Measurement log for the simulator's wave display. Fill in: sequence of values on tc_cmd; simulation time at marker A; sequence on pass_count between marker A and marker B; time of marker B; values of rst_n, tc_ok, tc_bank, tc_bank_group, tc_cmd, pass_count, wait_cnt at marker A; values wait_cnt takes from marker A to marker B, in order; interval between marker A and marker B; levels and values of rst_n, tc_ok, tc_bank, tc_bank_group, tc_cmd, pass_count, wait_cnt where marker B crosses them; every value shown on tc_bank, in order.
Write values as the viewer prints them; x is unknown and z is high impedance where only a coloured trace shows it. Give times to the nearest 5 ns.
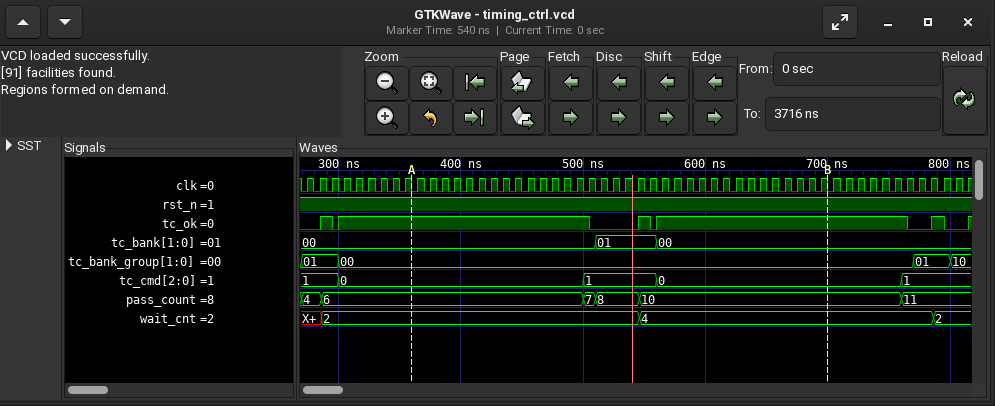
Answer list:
1, 0, 1, 0, 1
360 ns
6, 7, 8, 10
700 ns
rst_n=1, tc_ok=1, tc_bank=00, tc_bank_group=00, tc_cmd=0, pass_count=6, wait_cnt=2
2, 4
340 ns
rst_n=1, tc_ok=1, tc_bank=00, tc_bank_group=00, tc_cmd=0, pass_count=10, wait_cnt=4
00, 01, 00
